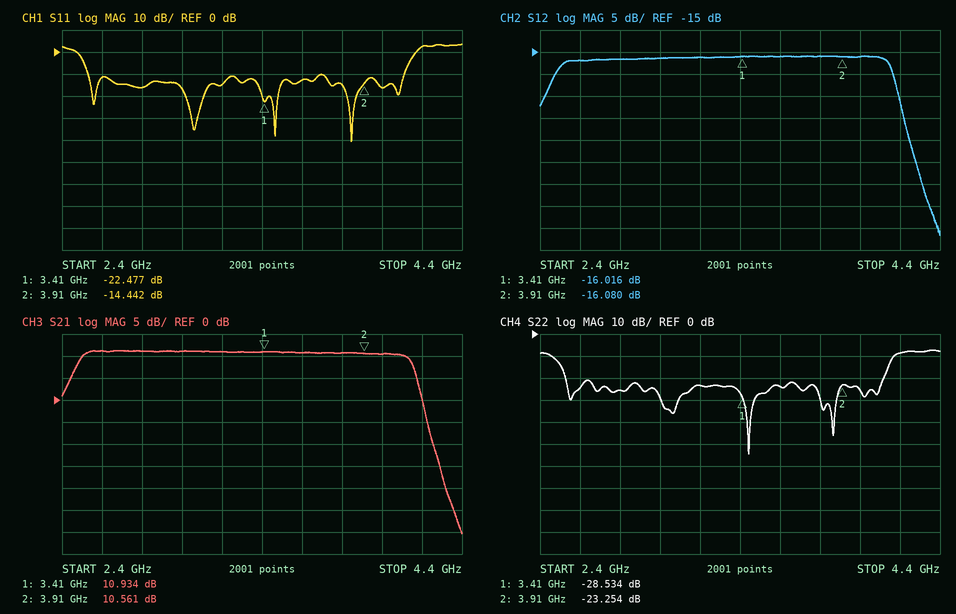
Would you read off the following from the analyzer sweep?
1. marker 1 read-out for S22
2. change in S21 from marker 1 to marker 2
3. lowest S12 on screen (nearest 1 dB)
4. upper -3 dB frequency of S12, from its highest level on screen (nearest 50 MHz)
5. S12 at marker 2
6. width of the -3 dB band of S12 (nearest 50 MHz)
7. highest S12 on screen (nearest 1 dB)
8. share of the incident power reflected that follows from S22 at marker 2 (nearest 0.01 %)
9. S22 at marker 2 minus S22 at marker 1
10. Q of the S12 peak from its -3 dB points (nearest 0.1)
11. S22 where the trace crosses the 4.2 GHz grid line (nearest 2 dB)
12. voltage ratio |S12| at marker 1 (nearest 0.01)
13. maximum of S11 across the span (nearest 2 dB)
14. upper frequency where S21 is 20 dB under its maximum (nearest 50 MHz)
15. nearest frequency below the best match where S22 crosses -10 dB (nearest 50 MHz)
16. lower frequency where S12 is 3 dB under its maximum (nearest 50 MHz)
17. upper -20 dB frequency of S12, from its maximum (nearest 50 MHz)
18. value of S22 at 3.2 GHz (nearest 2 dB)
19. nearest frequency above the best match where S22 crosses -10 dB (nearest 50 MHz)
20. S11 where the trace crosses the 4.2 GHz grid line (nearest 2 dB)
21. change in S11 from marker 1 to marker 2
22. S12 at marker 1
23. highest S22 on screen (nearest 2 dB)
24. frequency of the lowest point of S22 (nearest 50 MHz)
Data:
-28.534 dB
-0.373 dB
-57 dB
4.15 GHz
-16.080 dB
1.65 GHz
-16 dB
0.47 %
5.280 dB
2.0
-8 dB
0.16
4 dB
4.25 GHz
2.45 GHz
2.50 GHz
4.25 GHz
-24 dB
4.15 GHz
2 dB
8.035 dB
-16.016 dB
-8 dB
3.45 GHz
